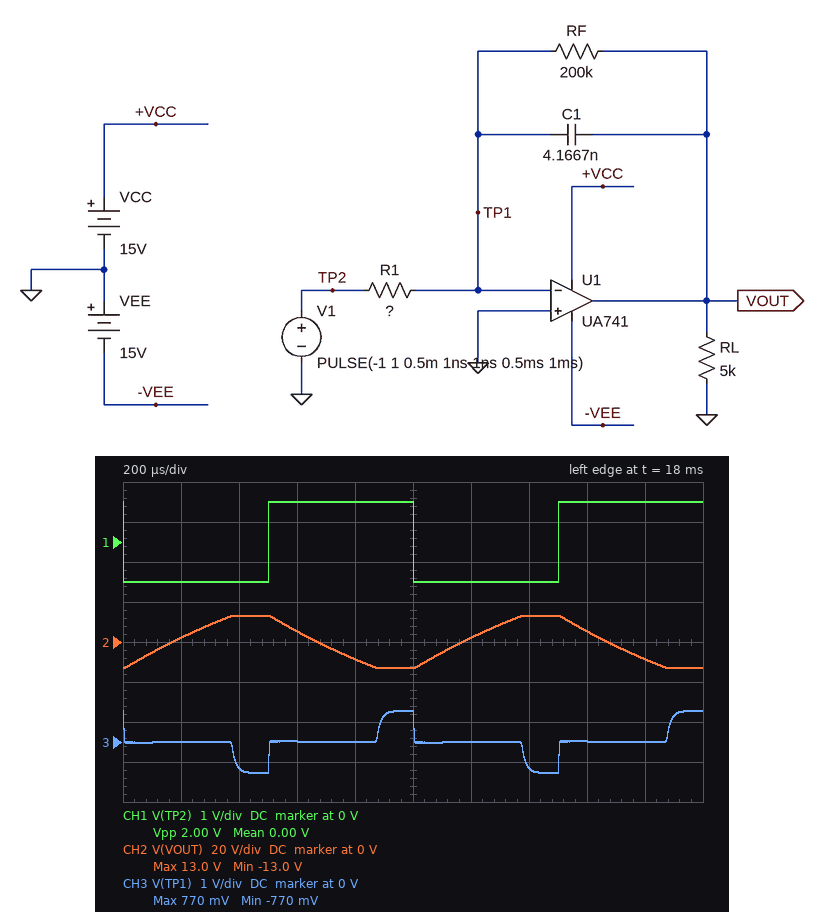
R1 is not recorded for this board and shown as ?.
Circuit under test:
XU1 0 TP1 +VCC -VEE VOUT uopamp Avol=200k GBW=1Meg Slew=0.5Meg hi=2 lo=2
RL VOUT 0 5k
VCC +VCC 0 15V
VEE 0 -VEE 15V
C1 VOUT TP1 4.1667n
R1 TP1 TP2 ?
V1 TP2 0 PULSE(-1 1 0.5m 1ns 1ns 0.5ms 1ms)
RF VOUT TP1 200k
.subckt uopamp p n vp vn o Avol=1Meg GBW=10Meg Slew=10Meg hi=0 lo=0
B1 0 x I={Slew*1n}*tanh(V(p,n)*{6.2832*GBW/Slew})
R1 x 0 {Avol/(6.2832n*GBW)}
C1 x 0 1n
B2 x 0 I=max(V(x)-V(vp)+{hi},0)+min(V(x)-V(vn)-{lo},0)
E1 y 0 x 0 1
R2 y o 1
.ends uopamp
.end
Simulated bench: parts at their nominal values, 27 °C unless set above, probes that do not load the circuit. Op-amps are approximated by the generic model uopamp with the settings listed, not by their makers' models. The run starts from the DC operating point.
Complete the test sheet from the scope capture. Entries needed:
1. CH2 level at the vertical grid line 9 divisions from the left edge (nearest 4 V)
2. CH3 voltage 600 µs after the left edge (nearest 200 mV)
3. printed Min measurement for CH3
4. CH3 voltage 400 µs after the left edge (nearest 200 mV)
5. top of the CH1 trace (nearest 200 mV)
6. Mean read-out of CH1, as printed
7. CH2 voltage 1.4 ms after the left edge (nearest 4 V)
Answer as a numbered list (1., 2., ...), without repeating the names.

1. -8 V
2. 0 V
3. -770 mV
4. -600 mV
5. 1.0 V
6. 0.00 V
7. 12 V
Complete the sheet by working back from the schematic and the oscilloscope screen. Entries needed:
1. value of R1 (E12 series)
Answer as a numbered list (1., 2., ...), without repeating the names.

1. 3.3 kΩ
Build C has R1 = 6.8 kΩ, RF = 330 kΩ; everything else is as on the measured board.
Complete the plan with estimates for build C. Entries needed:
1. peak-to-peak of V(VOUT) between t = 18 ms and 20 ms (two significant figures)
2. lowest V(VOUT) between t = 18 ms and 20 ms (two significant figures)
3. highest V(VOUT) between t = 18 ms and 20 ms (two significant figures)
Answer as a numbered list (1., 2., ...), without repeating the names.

1. 17 V
2. -8.7 V
3. 8.7 V
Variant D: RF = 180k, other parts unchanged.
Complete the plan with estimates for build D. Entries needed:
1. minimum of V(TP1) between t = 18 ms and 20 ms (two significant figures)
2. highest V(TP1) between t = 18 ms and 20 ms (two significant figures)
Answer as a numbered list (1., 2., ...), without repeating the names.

1. -750 mV
2. 750 mV
